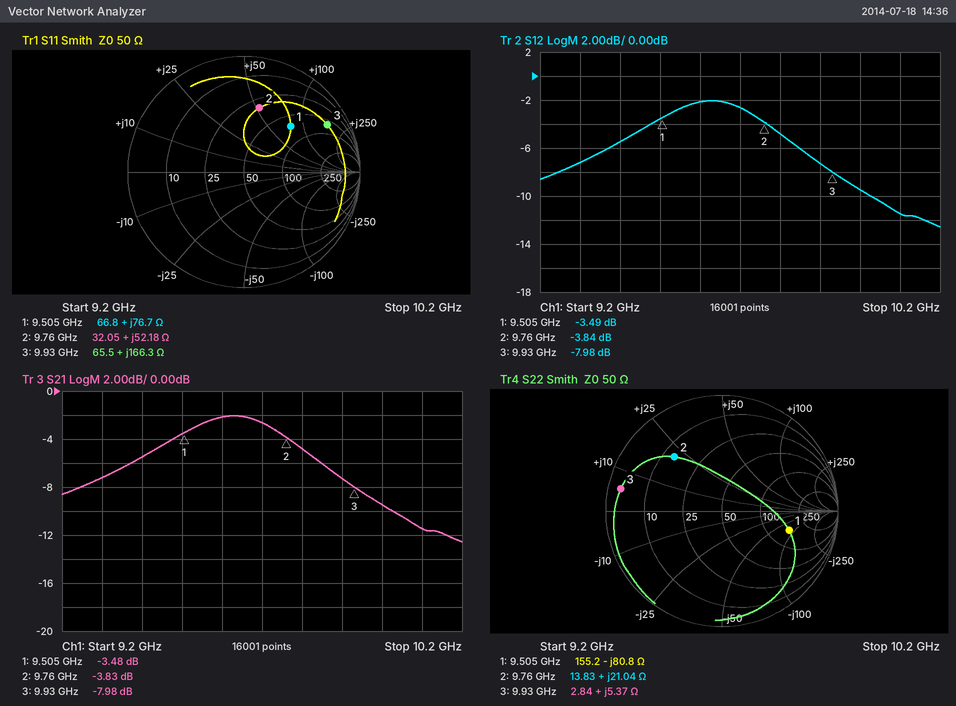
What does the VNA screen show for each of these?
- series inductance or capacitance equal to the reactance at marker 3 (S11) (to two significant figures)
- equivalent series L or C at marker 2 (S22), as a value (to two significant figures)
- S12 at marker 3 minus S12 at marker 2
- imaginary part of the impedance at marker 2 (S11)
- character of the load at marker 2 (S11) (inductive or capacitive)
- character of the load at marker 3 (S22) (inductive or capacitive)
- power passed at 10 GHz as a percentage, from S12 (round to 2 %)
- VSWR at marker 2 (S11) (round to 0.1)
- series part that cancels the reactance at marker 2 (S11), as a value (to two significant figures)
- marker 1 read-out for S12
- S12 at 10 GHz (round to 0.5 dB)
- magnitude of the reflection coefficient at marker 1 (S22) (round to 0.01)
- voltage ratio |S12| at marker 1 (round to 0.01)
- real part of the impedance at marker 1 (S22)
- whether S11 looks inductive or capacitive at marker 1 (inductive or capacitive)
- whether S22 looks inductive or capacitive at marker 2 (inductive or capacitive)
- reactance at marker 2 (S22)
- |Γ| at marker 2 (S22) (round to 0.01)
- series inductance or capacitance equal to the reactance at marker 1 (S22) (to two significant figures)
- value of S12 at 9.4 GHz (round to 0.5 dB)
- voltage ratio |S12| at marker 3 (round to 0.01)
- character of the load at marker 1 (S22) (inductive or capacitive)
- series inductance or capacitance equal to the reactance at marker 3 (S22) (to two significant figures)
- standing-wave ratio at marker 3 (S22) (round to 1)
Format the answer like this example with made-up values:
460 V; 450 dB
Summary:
2.7 nH; 340 pH; -4.14 dB; +52.18 Ω; inductive; inductive; 12 %; 3.6; 310 fF; -3.49 dB; -9.5 dB; 0.60; 0.67; 155.2 Ω; inductive; inductive; +21.04 Ω; 0.62; 210 fF; -5.5 dB; 0.40; capacitive; 86 pH; 18
